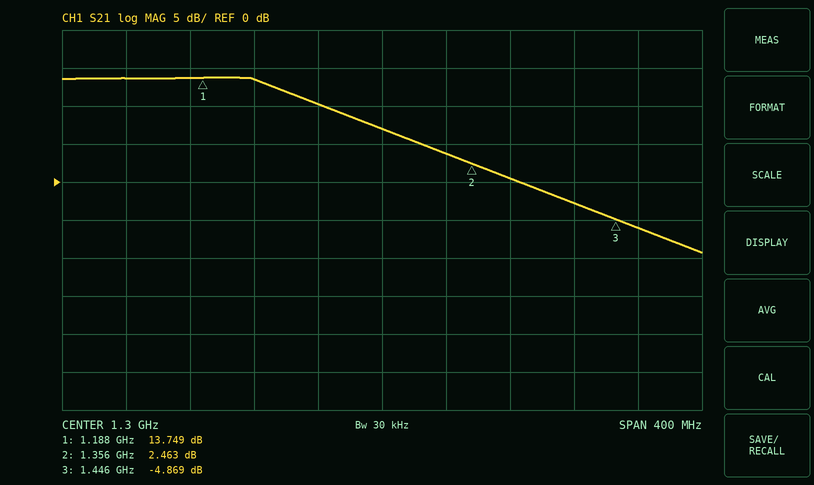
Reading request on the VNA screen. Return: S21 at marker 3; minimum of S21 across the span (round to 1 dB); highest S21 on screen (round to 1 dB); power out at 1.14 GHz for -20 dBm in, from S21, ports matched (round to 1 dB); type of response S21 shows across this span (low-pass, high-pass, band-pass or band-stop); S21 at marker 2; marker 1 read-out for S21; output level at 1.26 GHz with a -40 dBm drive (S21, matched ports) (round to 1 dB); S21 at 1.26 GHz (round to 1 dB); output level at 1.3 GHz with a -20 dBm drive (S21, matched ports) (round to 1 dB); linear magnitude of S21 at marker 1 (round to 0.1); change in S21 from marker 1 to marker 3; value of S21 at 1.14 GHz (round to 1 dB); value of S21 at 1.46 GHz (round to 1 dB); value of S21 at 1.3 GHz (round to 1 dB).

-4.869 dB
-9 dB
14 dB
-6 dBm
low-pass
2.463 dB
13.749 dB
-30 dBm
10 dB
-13 dBm
4.9
-18.618 dB
14 dB
-6 dB
7 dB
